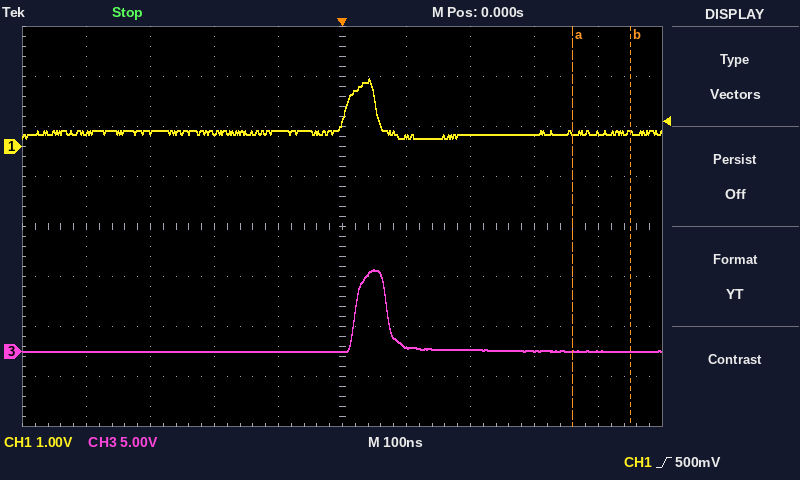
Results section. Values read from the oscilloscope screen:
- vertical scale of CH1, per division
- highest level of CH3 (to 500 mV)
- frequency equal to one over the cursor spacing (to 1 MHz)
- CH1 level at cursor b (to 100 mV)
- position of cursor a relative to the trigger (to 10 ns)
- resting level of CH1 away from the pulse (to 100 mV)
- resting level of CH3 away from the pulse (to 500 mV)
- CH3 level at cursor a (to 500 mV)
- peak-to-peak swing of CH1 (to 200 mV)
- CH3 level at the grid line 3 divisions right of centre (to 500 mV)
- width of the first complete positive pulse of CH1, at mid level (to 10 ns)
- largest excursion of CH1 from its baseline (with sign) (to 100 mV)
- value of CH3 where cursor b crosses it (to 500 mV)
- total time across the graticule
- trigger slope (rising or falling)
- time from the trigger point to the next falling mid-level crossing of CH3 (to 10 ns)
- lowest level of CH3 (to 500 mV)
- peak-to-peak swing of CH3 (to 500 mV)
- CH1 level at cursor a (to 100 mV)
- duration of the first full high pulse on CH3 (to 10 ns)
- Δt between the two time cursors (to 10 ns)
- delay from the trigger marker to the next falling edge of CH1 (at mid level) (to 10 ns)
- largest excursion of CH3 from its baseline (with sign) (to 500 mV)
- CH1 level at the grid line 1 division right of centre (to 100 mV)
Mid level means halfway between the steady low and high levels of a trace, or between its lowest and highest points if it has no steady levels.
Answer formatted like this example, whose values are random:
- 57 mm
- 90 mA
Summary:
- 1 V
- 8.0 V
- 11 MHz
- 300 mV
- +360 ns
- 300 mV
- 0.0 V
- 0.0 V
- 1.2 V
- 0.0 V
- 50 ns
- +1.1 V
- 0.0 V
- 1 µs
- rising
- 70 ns
- 0.0 V
- 8.0 V
- 300 mV
- 50 ns
- 90 ns
- 50 ns
- +8.0 V
- 200 mV
